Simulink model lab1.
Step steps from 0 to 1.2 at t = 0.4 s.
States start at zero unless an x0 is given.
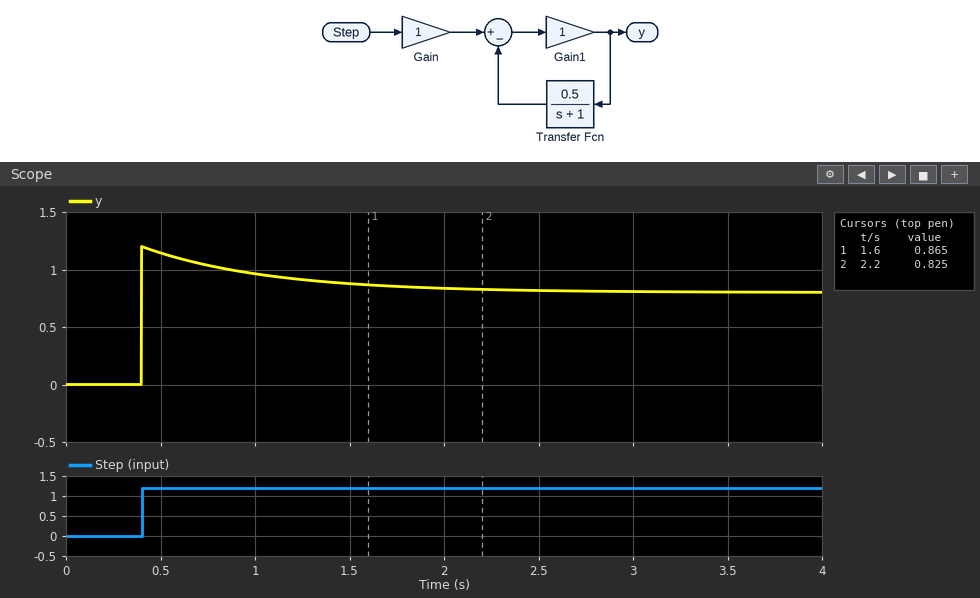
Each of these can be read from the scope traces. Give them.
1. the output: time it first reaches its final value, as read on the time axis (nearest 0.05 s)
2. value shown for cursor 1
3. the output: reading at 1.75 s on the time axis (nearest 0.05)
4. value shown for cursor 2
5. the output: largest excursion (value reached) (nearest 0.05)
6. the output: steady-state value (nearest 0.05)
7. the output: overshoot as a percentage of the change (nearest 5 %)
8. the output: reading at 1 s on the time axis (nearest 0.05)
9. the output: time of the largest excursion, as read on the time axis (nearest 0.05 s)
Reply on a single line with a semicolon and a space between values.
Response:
0.40 s; 0.865; 0.85; 0.825; 1.20; 0.80; 50 %; 0.95; 0.40 s
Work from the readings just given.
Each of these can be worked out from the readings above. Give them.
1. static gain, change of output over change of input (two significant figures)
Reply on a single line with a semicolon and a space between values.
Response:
0.67
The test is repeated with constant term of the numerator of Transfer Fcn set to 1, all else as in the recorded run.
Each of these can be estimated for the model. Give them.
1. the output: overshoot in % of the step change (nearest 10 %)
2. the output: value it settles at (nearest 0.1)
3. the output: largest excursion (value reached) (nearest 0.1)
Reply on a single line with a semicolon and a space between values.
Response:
100 %; 0.6; 1.2
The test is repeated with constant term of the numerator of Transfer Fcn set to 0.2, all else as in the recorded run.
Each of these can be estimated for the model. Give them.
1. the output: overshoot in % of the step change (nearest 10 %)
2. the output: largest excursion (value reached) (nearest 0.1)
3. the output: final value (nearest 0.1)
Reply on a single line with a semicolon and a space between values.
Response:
20 %; 1.2; 1.0
